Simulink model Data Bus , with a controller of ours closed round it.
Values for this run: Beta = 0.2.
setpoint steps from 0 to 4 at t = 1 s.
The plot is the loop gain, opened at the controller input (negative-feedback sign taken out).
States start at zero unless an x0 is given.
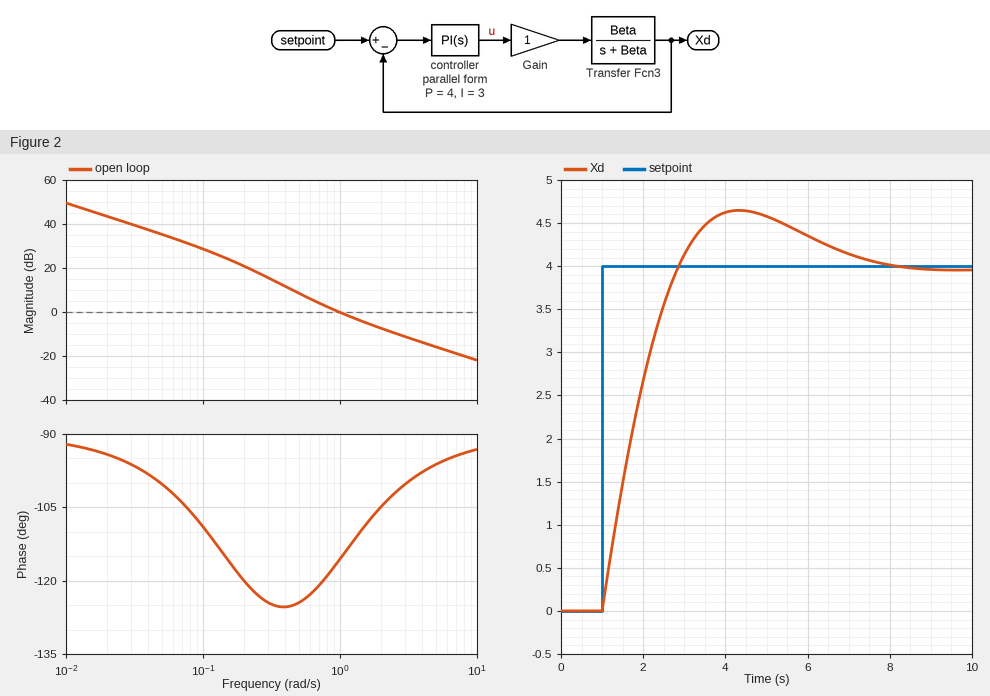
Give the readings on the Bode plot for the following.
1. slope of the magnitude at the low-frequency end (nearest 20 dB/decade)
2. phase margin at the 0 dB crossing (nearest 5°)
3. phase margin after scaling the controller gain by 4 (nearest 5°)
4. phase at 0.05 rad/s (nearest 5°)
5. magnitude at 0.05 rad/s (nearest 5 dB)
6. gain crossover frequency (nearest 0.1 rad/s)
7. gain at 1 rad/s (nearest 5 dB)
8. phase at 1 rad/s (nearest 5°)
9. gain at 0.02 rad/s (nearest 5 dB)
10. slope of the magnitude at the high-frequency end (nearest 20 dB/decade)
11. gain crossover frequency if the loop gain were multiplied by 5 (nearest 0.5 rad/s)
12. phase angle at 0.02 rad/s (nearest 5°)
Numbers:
-20 dB/decade
65°
80°
-100°
35 dB
1.0 rad/s
0 dB
-115°
45 dB
-20 dB/decade
4.0 rad/s
-95°
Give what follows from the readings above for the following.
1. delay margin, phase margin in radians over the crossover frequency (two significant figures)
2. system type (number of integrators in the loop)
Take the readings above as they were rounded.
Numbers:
1.1 s
1
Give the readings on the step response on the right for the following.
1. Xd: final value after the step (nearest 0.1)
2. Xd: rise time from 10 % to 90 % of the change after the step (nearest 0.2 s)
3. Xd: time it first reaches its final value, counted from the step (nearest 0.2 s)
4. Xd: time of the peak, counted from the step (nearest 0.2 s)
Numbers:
4.0
1.4 s
1.8 s
3.4 s
